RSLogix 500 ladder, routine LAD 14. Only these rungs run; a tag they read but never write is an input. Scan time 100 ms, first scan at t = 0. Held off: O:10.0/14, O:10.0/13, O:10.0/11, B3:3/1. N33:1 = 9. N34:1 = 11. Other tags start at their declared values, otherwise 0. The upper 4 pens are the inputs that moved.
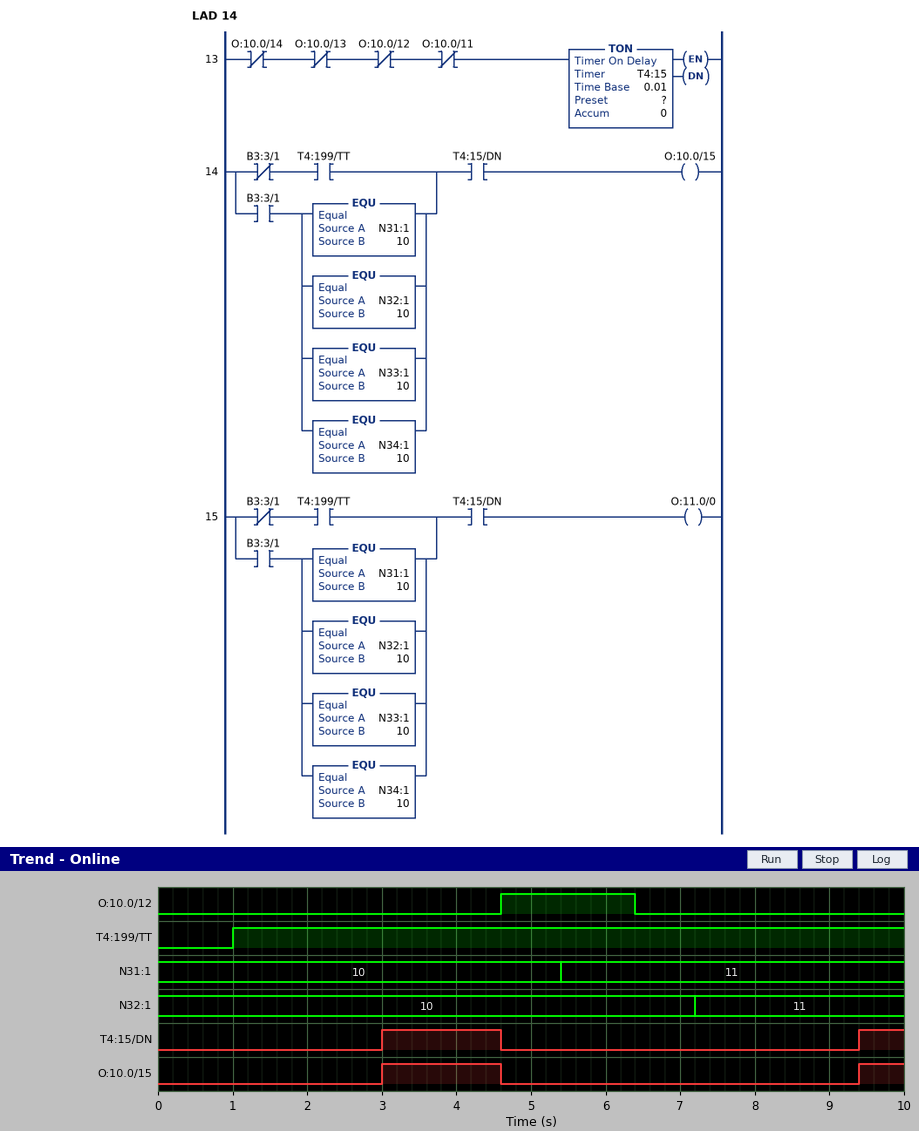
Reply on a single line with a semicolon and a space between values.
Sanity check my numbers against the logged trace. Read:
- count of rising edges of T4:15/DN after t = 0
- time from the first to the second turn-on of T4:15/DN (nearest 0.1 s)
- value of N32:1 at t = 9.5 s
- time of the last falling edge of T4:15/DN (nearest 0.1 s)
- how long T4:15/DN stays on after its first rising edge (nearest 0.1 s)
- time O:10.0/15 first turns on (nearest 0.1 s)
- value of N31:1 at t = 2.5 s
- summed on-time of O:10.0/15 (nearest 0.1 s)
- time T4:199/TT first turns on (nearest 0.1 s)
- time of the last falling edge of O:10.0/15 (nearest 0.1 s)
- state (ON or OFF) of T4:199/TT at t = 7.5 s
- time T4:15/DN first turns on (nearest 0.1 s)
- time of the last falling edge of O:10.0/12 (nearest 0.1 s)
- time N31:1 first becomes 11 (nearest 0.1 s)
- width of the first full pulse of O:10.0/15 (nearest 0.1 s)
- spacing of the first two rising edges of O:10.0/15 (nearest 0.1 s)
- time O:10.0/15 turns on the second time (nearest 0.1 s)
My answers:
2; 6.4 s; 11; 4.6 s; 1.6 s; 3.0 s; 10; 2.2 s; 1.0 s; 4.6 s; ON; 3.0 s; 6.4 s; 5.4 s; 1.6 s; 6.4 s; 9.4 s
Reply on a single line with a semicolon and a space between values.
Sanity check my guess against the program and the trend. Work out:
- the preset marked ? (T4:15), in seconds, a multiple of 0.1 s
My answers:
3.0 s
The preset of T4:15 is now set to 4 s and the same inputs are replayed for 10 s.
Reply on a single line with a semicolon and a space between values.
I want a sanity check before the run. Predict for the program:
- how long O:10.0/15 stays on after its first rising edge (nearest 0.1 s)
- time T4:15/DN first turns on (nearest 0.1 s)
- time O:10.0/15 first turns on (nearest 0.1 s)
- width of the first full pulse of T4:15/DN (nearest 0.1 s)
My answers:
0.6 s; 4.0 s; 4.0 s; 0.6 s
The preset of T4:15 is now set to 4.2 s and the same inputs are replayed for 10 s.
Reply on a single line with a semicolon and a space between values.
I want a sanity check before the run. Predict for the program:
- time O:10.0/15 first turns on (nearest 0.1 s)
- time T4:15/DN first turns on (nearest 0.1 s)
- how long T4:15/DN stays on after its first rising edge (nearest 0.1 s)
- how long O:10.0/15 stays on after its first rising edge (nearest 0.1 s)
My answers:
4.2 s; 4.2 s; 0.4 s; 0.4 s
